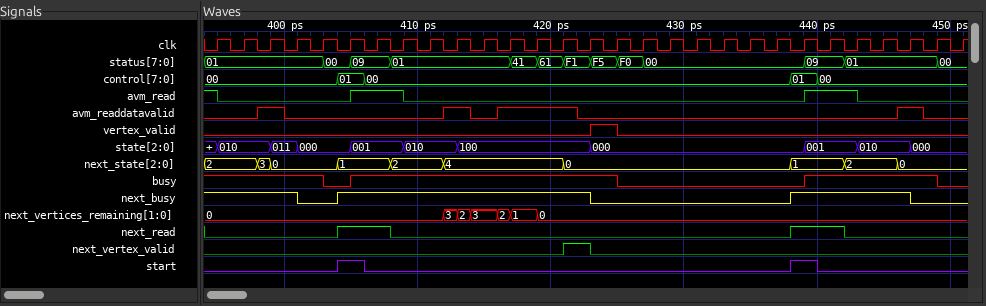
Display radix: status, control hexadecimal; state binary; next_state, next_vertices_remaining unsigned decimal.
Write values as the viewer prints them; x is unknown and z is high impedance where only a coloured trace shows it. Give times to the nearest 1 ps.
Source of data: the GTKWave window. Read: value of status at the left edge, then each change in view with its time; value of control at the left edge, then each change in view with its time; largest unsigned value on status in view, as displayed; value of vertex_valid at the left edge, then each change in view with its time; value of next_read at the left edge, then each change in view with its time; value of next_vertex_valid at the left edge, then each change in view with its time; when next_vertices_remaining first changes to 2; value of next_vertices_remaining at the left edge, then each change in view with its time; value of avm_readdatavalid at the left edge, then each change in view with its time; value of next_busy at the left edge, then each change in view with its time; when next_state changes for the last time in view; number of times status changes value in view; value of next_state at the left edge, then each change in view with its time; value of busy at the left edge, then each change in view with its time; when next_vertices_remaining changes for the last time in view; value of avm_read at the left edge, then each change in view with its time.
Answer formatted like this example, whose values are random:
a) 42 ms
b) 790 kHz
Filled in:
a) 01, 00 at 403 ps, 09 at 405 ps, 01 at 408 ps, 41 at 417 ps, 61 at 419 ps, F1 at 421 ps, F5 at 423 ps, F0 at 425 ps, 00 at 427 ps, 09 at 439 ps, 01 at 442 ps, 00 at 449 ps
b) 00, 01 at 404 ps, 00 at 406 ps, 01 at 438 ps, 00 at 440 ps
c) F5
d) 0, 1 at 423 ps, 0 at 425 ps
e) 0, 1 at 404 ps, 0 at 408 ps, 1 at 438 ps, 0 at 442 ps
f) 0, 1 at 421 ps, 0 at 423 ps
g) 413 ps
h) 0, 3 at 412 ps, 2 at 413 ps, 3 at 414 ps, 2 at 416 ps, 1 at 417 ps, 0 at 419 ps
i) 0, 1 at 398 ps, 0 at 400 ps, 1 at 412 ps, 0 at 414 ps, 1 at 416 ps, 0 at 422 ps, 1 at 446 ps, 0 at 448 ps
j) 1, 0 at 401 ps, 1 at 404 ps, 0 at 423 ps, 1 at 438 ps, 0 at 447 ps
k) 446 ps
l) 12
m) 2, 3 at 398 ps, 0 at 399 ps, 1 at 404 ps, 2 at 408 ps, 4 at 412 ps, 0 at 421 ps, 1 at 438 ps, 2 at 442 ps, 0 at 446 ps
n) 1, 0 at 403 ps, 1 at 405 ps, 0 at 425 ps, 1 at 439 ps, 0 at 449 ps
o) 419 ps
p) 1, 0 at 395 ps, 1 at 405 ps, 0 at 409 ps, 1 at 439 ps, 0 at 443 ps
